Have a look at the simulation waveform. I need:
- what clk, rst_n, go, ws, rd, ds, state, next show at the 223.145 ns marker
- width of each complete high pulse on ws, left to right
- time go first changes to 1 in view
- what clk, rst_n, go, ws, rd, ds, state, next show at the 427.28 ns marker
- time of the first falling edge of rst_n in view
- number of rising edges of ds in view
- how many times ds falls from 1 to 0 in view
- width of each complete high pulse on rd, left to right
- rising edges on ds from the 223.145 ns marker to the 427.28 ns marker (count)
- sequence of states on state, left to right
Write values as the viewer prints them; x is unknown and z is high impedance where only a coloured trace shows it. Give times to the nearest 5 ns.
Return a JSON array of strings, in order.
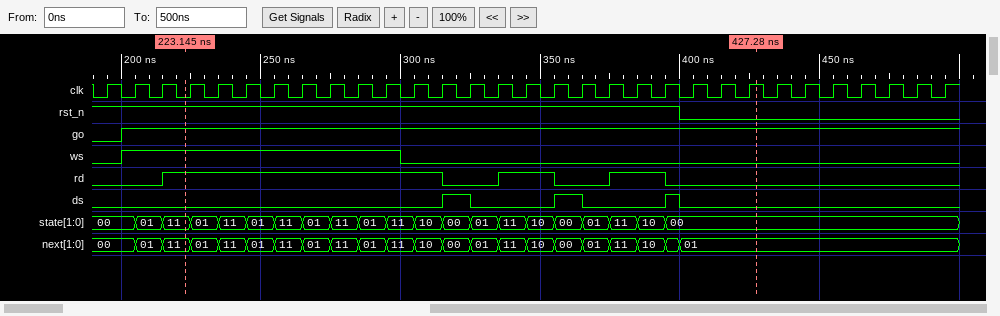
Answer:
["clk=0, rst_n=1, go=1, ws=1, rd=1, ds=0, state=11, next=11", "100 ns", "200 ns", "clk=1, rst_n=0, go=1, ws=0, rd=0, ds=0, state=00, next=01", "400 ns", "3", "3", "100 ns, 20 ns, 20 ns", "3", "00, 01, 11, 01, 11, 01, 11, 01, 11, 01, 11, 10, 00, 01, 11, 10, 00, 01, 11, 10, 00"]
